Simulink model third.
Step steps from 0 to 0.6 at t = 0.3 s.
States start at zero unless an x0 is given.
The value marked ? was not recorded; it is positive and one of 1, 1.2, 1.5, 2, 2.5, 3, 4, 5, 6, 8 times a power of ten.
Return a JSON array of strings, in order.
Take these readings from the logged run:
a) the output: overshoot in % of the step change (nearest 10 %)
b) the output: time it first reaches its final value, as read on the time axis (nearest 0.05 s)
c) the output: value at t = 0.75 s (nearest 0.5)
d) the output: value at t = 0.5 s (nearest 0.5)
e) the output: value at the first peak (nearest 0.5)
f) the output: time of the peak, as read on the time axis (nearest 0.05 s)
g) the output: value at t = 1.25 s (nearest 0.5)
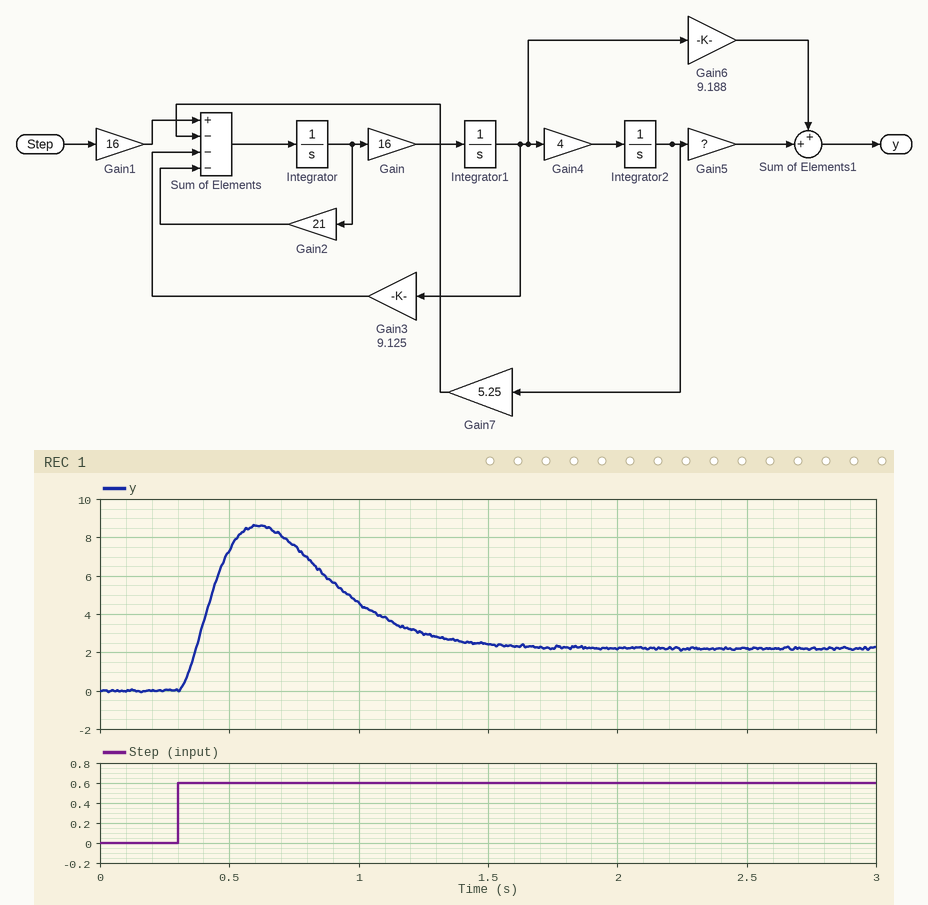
["290 %", "0.35 s", "7.5", "7.5", "8.5", "0.60 s", "3.0"]
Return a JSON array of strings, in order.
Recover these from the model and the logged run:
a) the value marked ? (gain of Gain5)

["1.2"]
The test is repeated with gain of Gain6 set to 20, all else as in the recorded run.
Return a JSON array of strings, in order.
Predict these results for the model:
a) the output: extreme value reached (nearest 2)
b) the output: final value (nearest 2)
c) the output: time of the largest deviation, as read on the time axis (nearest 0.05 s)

["18", "2", "0.60 s"]
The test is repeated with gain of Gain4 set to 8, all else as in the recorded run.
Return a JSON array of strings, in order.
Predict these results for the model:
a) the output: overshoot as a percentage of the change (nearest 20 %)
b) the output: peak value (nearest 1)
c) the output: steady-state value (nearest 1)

["280 %", "8", "2"]
